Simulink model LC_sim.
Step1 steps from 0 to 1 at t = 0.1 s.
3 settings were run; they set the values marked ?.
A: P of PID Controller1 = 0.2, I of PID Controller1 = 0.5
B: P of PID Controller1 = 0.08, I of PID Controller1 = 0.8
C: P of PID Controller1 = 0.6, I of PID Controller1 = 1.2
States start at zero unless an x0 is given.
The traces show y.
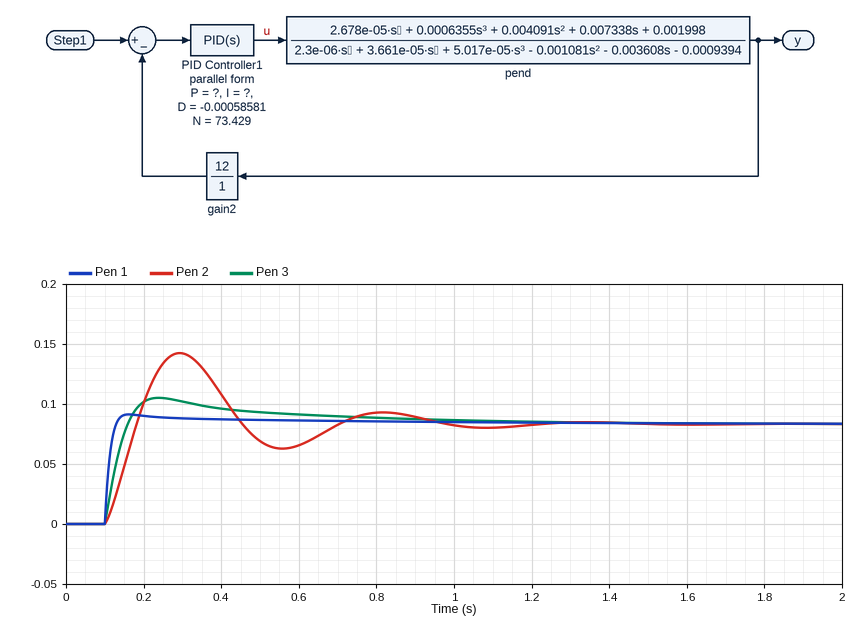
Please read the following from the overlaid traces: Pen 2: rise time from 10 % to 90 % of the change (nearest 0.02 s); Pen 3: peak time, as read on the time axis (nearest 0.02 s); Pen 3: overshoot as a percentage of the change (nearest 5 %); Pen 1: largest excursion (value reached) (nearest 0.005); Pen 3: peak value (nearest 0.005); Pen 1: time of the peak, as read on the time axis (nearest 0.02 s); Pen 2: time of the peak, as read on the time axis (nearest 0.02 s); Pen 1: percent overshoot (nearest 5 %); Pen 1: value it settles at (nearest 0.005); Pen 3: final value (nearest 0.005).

0.06 s
0.24 s
25 %
0.090
0.105
0.16 s
0.30 s
10 %
0.085
0.085
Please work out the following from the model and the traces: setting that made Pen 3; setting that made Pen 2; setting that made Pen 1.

A
B
C
